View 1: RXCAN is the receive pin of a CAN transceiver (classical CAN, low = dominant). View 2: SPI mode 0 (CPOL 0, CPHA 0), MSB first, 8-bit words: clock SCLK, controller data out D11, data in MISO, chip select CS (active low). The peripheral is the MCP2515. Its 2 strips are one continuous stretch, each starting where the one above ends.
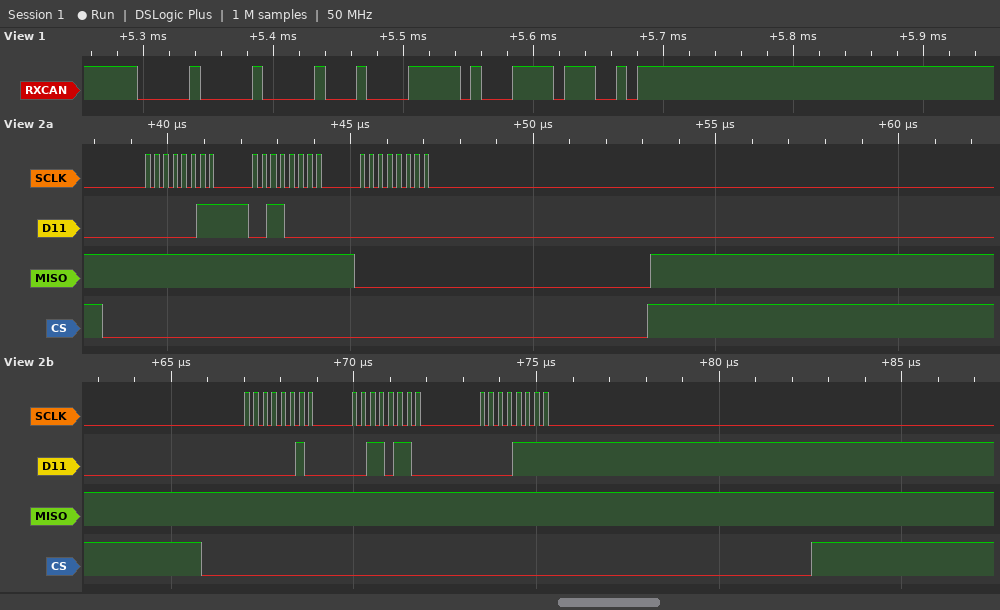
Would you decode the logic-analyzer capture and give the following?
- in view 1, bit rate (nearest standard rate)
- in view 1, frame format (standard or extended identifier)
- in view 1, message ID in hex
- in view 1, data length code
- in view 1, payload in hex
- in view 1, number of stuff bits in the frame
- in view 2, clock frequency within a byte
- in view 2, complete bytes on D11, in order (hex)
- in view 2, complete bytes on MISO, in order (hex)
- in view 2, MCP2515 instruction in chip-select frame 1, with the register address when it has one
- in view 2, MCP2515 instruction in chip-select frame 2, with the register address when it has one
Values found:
125 kbit/s
standard
0x000
1
0F
4
4 MHz
0x03 0x30 0x00 0x02 0x36 0x0F
0xFF 0xFF 0x00 0xFF 0xFF 0xFF
READ 0x30
WRITE 0x36
